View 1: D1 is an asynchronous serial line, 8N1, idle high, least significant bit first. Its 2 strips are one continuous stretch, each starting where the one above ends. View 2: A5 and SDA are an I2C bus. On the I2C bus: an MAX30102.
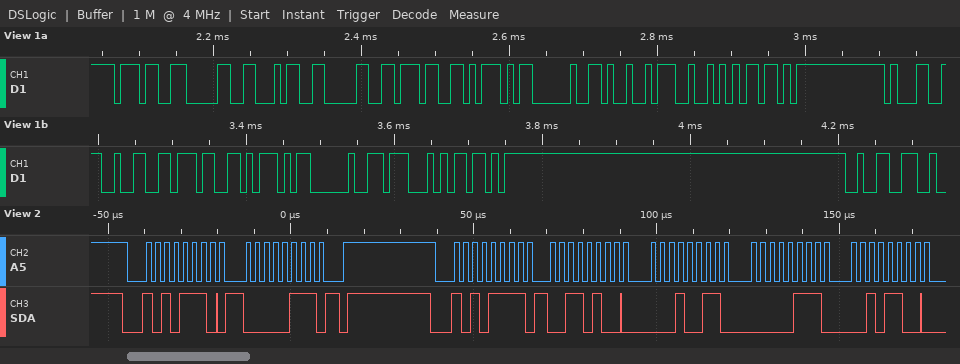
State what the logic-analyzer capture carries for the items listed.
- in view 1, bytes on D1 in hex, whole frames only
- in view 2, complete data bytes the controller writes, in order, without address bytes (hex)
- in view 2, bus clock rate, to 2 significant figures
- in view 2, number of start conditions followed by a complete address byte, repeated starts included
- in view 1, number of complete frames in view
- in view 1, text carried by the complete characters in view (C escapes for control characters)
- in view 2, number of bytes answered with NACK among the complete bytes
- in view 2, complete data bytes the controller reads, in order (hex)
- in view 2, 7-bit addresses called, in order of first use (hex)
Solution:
37 30 34 30 37 5D 20 49 52 5B 31 32 37 5D 20 47 5B 32
07
400 kHz
2
18
"70407] IR[127] G[2"
0
34 13 07 2C
0x57
